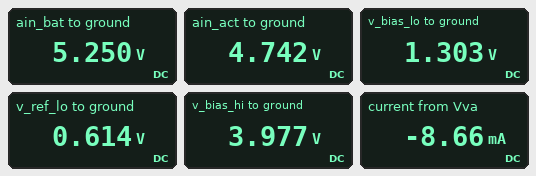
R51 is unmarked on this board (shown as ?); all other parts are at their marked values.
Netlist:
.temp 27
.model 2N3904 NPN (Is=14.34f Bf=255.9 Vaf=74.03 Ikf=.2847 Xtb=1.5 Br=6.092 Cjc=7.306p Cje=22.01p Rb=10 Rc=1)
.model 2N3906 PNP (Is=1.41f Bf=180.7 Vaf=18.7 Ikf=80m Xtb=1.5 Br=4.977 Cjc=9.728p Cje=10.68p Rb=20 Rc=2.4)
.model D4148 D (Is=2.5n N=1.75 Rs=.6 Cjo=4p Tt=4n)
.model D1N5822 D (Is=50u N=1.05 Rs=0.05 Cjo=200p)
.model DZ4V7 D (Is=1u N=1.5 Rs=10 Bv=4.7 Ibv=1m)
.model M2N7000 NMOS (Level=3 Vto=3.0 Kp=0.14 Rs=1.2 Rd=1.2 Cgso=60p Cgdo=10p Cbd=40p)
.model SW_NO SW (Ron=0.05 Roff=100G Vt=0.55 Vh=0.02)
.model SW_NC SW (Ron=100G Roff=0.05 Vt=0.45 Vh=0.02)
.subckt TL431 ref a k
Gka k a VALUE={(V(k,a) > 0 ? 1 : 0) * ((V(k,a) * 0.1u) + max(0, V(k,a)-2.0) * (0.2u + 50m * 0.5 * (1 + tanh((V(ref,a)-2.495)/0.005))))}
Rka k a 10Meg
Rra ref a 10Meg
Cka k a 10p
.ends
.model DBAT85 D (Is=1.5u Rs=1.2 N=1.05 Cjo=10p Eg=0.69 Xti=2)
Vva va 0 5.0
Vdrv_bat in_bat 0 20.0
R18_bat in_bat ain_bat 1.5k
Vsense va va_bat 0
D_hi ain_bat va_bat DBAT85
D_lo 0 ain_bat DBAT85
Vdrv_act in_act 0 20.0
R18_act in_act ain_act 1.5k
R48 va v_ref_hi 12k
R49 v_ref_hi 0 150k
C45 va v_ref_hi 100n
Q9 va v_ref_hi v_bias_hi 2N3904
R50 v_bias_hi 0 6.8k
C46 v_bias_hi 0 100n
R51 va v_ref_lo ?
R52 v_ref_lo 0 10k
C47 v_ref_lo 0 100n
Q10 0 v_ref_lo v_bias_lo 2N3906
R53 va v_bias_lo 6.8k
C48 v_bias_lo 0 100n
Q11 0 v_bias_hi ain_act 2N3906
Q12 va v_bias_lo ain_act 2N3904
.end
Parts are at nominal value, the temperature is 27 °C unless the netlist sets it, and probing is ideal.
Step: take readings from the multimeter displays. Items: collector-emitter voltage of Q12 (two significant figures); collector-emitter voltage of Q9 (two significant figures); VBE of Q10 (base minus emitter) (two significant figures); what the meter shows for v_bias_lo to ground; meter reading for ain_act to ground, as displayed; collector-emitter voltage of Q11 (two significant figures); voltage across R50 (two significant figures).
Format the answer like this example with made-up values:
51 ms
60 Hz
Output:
260 mV
1.0 V
-690 mV
1.303 V
4.742 V
-4.7 V
4.0 V
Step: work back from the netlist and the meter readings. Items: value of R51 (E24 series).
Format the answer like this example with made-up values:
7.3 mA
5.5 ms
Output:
75 kΩ
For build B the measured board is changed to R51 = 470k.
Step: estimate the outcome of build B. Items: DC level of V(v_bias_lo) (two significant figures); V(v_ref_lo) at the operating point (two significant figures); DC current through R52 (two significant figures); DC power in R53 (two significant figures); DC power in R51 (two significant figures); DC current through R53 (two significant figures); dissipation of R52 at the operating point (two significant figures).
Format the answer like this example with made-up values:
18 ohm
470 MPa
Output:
830 mV
140 mV
14 µA
2.6 mW
50 µW
610 µA
1.9 µW
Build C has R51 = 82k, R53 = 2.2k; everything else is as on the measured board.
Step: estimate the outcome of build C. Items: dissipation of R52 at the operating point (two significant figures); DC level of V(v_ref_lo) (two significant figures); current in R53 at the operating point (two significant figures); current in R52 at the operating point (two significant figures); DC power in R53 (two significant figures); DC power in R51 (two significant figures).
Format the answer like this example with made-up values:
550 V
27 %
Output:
39 µW
620 mV
1.7 mA
62 µA
6.1 mW
230 µW
